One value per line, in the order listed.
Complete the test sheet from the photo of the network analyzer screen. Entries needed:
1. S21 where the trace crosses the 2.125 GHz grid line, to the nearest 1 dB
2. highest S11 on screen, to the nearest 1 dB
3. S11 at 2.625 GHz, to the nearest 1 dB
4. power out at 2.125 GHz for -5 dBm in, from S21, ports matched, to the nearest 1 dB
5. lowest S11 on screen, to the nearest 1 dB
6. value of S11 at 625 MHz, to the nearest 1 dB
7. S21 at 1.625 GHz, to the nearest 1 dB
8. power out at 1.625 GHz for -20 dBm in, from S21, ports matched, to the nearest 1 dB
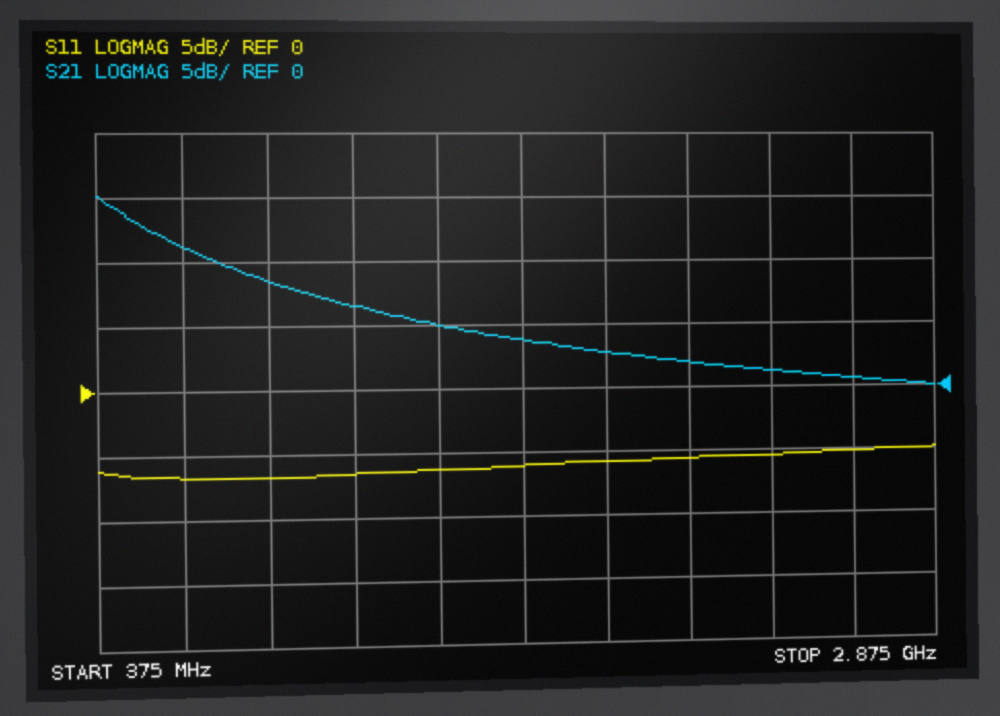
2 dB
-5 dB
-5 dB
-3 dBm
-7 dB
-7 dB
4 dB
-16 dBm
